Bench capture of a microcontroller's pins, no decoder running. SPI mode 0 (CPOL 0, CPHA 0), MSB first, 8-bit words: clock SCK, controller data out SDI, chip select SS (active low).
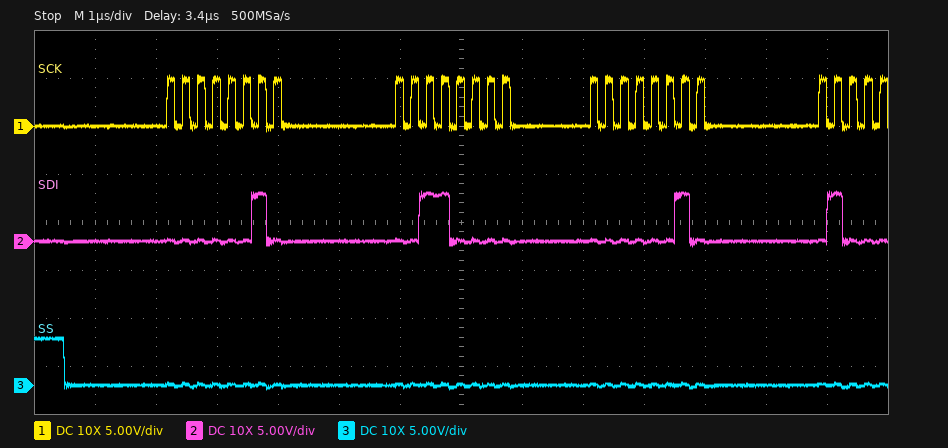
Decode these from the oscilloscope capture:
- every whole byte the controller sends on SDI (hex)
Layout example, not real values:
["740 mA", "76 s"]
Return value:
["02 30 02"]
